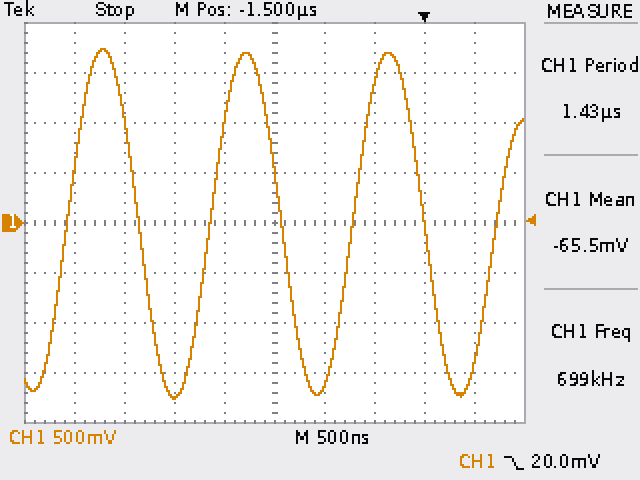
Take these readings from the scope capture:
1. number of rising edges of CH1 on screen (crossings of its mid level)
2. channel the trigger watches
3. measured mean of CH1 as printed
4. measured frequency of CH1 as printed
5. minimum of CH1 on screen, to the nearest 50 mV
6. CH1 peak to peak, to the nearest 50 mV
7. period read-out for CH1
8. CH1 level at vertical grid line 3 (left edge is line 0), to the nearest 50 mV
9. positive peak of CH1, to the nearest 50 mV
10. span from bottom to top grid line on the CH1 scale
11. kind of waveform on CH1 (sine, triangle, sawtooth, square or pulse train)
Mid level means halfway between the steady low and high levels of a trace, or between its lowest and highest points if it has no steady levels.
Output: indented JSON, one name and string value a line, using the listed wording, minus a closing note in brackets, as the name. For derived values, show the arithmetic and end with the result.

{
  "number of rising edges of CH1 on screen": "4",
  "channel the trigger watches": "CH1",
  "measured mean of CH1 as printed": "-65.5 mV",
  "measured frequency of CH1 as printed": "699 kHz",
  "minimum of CH1 on screen, to the nearest 50 mV": "-1.75 V",
  "CH1 peak to peak, to the nearest 50 mV": "1.75 V − (-1.75 V) = 3.50 V",
  "period read-out for CH1": "1.43 µs",
  "CH1 level at vertical grid line 3 (left edge is line 0), to the nearest 50 mV": "-1.75 V",
  "positive peak of CH1, to the nearest 50 mV": "1.75 V",
  "span from bottom to top grid line on the CH1 scale": "4 V",
  "kind of waveform on CH1": "sine"
}
